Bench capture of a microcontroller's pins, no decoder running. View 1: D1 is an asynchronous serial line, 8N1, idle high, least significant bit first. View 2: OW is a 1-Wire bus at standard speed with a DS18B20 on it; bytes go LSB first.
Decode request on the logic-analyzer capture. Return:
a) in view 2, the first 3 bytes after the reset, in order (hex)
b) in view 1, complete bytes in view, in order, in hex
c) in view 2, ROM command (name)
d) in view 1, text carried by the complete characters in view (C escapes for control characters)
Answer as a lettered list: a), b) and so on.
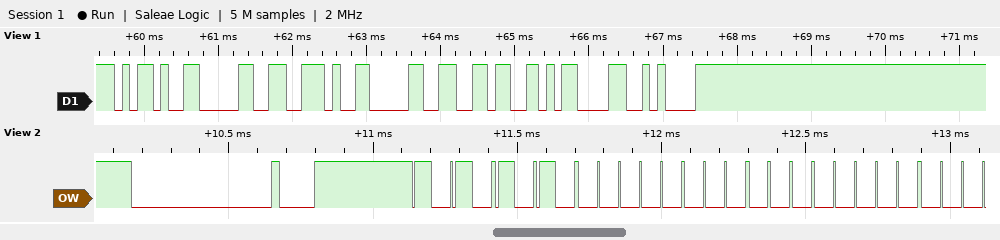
a) 55 00 00
b) 2D 30 2E 30 36 0D 0A
c) Match ROM
d) "-0.06\r\n"
